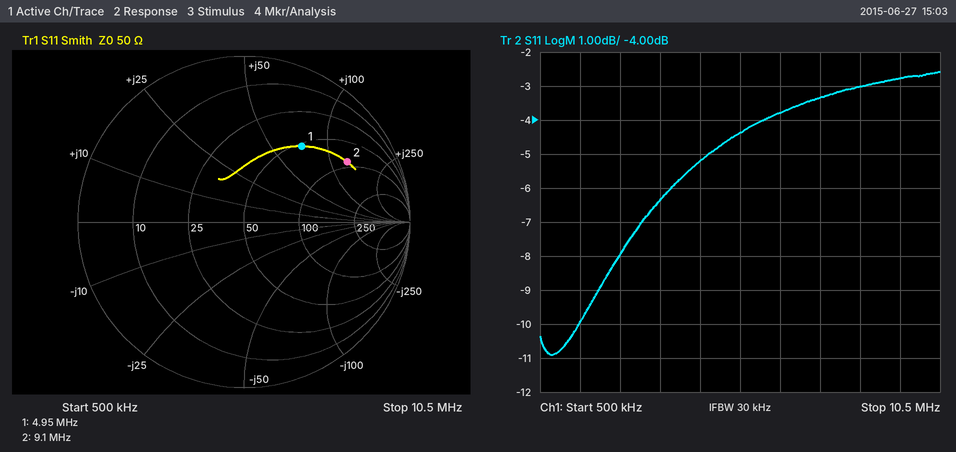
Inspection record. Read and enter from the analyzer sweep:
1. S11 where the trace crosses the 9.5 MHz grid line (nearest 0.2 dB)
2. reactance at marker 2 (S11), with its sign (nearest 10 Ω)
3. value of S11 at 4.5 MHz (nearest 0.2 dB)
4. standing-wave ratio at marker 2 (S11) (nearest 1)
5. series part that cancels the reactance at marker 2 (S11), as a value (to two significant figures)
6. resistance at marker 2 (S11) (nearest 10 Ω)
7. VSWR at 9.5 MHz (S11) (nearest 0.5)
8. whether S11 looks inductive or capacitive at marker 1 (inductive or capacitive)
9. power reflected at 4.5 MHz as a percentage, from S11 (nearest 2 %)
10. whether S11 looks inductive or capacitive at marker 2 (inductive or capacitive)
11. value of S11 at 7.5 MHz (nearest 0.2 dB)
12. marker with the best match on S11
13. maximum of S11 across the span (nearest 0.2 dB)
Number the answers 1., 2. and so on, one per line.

1. -2.8 dB
2. +130 Ω
3. -5.2 dB
4. 6
5. 130 pF
6. 90 Ω
7. 6.5
8. inductive
9. 30 %
10. inductive
11. -3.4 dB
12. marker 1
13. -2.6 dB
